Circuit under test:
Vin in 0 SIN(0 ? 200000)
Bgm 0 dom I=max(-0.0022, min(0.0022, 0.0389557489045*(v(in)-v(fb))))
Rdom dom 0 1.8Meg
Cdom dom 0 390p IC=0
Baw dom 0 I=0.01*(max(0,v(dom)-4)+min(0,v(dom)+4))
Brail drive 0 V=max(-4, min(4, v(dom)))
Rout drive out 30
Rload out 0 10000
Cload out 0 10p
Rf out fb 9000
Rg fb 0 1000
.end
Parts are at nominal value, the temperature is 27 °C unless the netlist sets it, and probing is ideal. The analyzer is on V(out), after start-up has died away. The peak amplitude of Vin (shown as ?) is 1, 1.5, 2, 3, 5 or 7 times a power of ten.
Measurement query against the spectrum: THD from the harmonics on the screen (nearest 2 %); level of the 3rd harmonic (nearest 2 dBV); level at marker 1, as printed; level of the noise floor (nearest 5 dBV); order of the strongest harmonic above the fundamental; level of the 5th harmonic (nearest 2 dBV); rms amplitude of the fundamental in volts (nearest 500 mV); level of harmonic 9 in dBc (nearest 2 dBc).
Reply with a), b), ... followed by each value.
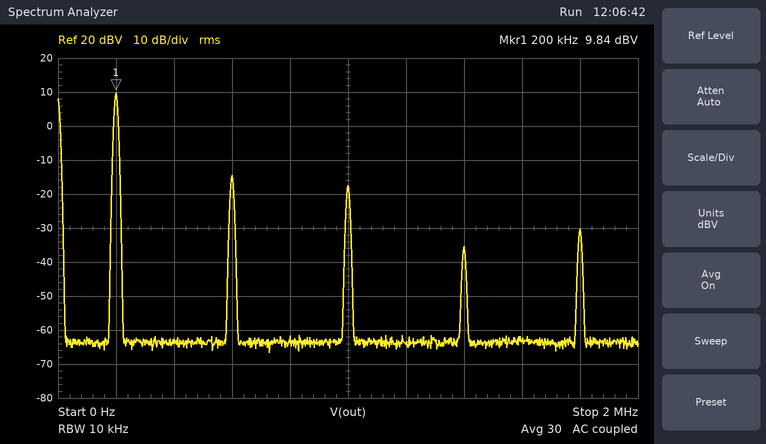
a) 8 %
b) -14 dBV
c) 9.84 dBV
d) -65 dBV
e) 3
f) -18 dBV
g) 3.0 V
h) -40 dBc
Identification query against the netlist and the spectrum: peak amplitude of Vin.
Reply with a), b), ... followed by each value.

a) 500 mV
